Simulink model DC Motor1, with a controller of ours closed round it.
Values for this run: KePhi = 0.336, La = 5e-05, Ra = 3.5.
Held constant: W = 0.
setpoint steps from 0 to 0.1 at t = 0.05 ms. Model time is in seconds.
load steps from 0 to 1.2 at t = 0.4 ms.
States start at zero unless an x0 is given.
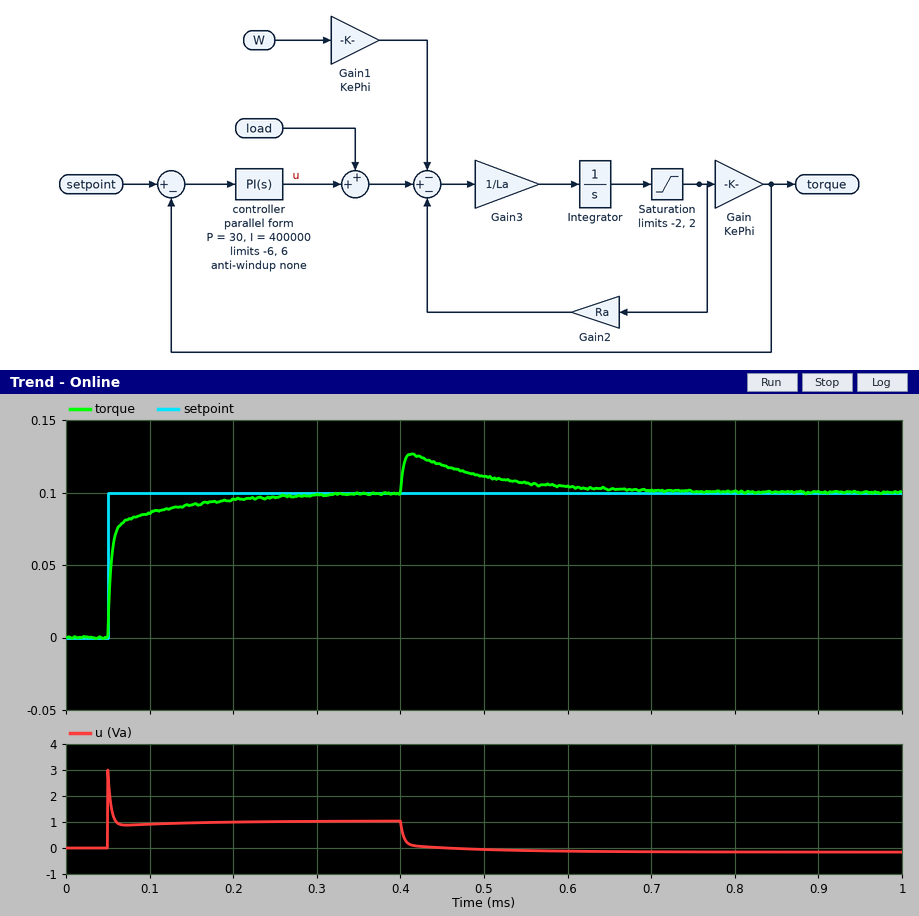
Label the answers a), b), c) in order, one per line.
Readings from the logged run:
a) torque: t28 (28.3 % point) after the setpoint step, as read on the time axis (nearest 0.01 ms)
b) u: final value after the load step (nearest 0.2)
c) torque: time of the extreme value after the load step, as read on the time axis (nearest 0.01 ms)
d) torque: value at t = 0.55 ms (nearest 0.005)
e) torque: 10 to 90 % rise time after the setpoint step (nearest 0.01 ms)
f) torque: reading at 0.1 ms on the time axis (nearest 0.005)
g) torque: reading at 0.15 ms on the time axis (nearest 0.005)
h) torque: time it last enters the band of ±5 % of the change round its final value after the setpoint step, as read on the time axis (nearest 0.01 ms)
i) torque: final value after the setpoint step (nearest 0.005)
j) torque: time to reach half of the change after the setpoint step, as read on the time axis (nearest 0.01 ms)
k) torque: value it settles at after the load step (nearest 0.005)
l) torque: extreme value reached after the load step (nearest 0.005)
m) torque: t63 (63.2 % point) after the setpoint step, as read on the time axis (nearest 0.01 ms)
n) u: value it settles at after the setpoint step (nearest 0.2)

a) 0.05 ms
b) -0.2
c) 0.41 ms
d) 0.105
e) 0.08 ms
f) 0.085
g) 0.090
h) 0.20 ms
i) 0.100
j) 0.05 ms
k) 0.100
l) 0.125
m) 0.06 ms
n) 1.0
